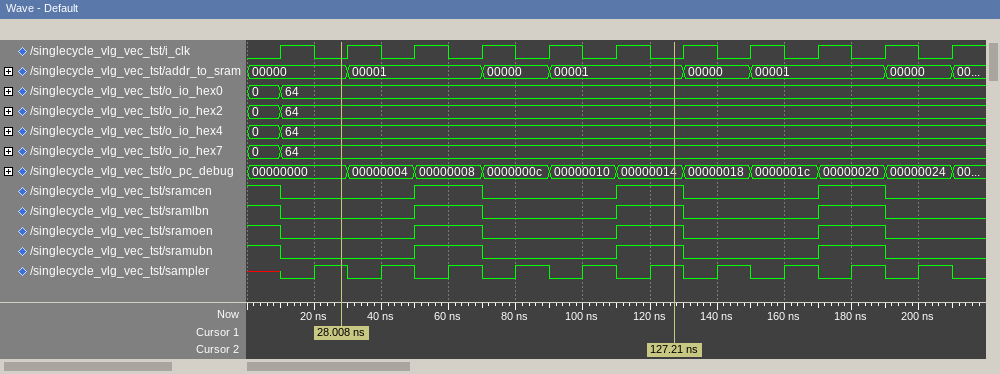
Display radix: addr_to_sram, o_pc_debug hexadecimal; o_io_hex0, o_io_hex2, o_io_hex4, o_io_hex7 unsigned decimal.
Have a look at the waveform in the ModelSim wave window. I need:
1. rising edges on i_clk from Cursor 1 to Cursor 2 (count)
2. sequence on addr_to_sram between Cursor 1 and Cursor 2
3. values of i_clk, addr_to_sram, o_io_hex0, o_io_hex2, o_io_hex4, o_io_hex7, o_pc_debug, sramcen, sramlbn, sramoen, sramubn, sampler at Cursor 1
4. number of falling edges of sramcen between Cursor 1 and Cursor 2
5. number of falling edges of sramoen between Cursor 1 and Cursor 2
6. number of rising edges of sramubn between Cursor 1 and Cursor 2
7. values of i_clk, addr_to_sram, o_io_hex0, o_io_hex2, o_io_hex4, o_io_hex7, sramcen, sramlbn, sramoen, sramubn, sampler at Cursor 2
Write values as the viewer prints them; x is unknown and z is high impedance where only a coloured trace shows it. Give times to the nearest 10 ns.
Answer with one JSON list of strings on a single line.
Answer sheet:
["5", "00000, 00001, 00000, 00001", "i_clk=0, addr_to_sram=00000, o_io_hex0=64, o_io_hex2=64, o_io_hex4=64, o_io_hex7=64, o_pc_debug=00000000, sramcen=0, sramlbn=0, sramoen=0, sramubn=0, sampler=1", "1", "1", "2", "i_clk=0, addr_to_sram=00001, o_io_hex0=64, o_io_hex2=64, o_io_hex4=64, o_io_hex7=64, sramcen=1, sramlbn=1, sramoen=1, sramubn=1, sampler=1"]
